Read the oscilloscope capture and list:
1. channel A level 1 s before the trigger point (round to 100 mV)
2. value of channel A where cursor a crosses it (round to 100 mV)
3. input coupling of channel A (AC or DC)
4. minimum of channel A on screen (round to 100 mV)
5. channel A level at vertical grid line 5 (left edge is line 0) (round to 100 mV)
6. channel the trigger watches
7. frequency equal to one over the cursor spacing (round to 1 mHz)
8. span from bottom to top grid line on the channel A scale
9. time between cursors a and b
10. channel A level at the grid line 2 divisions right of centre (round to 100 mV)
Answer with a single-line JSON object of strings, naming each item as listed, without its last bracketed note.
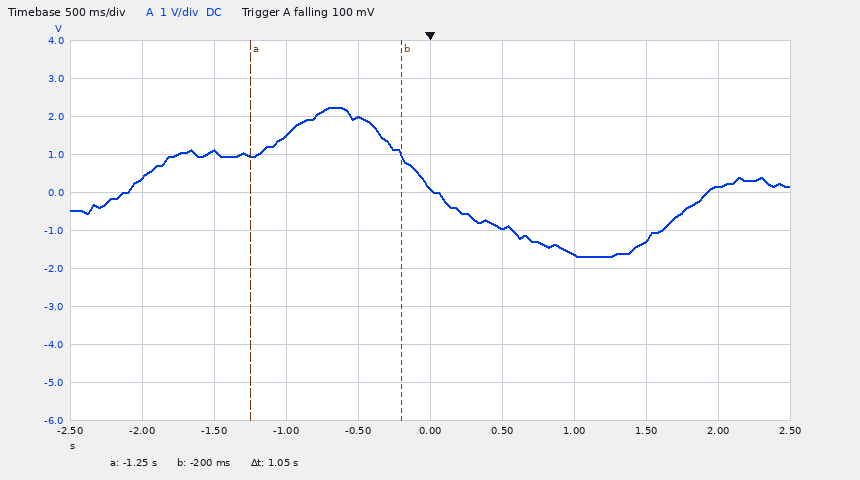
{"channel A level 1 s before the trigger point": "1.5 V", "value of channel A where cursor a crosses it": "1.0 V", "input coupling of channel A": "DC", "minimum of channel A on screen": "-1.7 V", "channel A level at vertical grid line 5 (left edge is line 0)": "100 mV", "channel the trigger watches": "channel A", "frequency equal to one over the cursor spacing": "952 mHz", "span from bottom to top grid line on the channel A scale": "10 V", "time between cursors a and b": "1.05 s", "channel A level at the grid line 2 divisions right of centre": "-1.6 V"}
